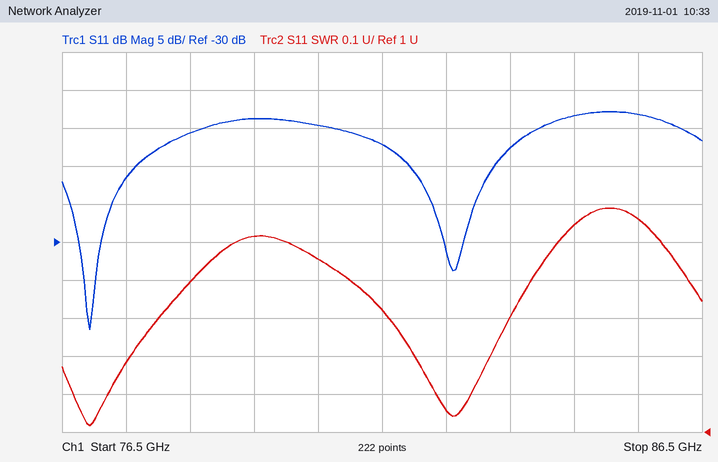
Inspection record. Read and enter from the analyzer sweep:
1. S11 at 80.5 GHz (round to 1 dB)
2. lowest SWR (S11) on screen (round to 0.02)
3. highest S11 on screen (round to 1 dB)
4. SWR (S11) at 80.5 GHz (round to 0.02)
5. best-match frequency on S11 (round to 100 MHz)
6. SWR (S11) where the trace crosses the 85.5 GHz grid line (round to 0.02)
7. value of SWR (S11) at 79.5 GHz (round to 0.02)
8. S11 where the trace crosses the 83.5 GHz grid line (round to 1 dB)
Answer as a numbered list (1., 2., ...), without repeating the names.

1. -15 dB
2. 1.02
3. -13 dB
4. 1.46
5. 76.9 GHz
6. 1.56
7. 1.52
8. -18 dB
